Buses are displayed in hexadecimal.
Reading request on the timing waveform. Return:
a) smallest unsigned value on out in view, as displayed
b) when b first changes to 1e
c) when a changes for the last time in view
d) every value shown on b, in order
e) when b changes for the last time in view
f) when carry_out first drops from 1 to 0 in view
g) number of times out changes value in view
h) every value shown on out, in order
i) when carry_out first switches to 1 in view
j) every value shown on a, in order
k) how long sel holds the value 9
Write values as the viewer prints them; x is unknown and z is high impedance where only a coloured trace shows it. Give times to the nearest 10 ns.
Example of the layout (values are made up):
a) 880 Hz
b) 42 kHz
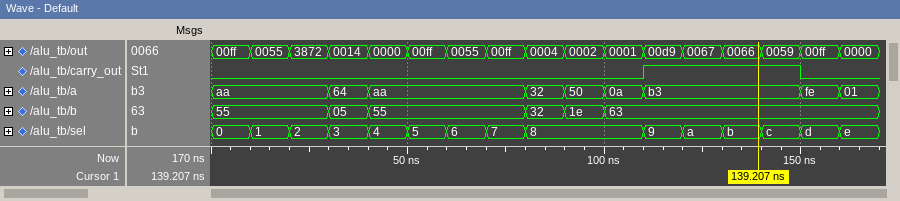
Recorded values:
a) 0000
b) 90 ns
c) 160 ns
d) 55, 05, 55, 32, 1e, 63
e) 100 ns
f) 150 ns
g) 16
h) 00ff, 0055, 3872, 0014, 0000, 00ff, 0055, 00ff, 0004, 0002, 0001, 00d9, 0067, 0066, 0059, 00ff, 0000
i) 110 ns
j) aa, 64, aa, 32, 50, 0a, b3, fe, 01
k) 10 ns
